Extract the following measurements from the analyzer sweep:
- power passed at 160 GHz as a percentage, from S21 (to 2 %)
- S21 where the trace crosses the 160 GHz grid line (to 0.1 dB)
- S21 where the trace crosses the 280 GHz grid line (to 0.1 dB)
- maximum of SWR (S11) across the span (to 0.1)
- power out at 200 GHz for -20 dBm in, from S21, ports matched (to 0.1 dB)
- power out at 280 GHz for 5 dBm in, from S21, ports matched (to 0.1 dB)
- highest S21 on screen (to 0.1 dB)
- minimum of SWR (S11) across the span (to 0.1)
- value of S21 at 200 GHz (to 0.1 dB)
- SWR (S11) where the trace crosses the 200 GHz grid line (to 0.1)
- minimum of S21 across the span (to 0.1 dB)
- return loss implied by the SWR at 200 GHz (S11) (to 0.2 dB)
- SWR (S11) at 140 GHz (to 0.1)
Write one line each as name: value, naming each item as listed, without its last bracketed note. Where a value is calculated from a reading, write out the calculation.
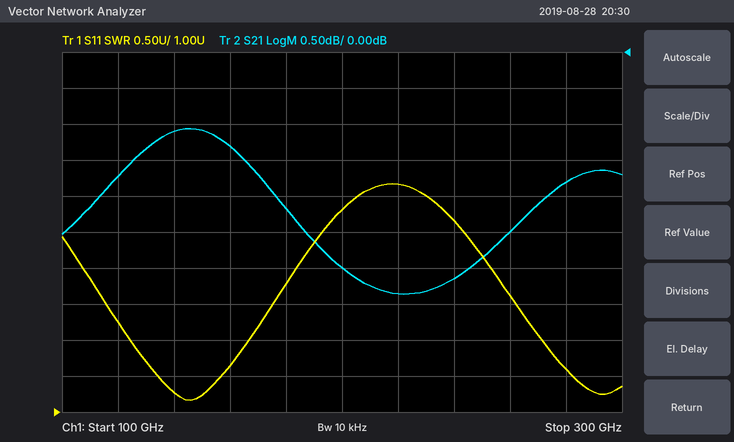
power passed at 160 GHz as a percentage, from S21: 10^(-1.3/10) ≈ 74 %
S21 where the trace crosses the 160 GHz grid line: -1.3 dB
S21 where the trace crosses the 280 GHz grid line: -1.8 dB
maximum of SWR (S11) across the span: 4.2
power out at 200 GHz for -20 dBm in, from S21, ports matched: -20 dBm + (-3.0 dB) = -23.0 dBm
power out at 280 GHz for 5 dBm in, from S21, ports matched: 5 dBm + (-1.8 dB) = 3.2 dBm
highest S21 on screen: -1.1 dB
minimum of SWR (S11) across the span: 1.2
value of S21 at 200 GHz: -3.0 dB
SWR (S11) where the trace crosses the 200 GHz grid line: 3.8
minimum of S21 across the span: -3.4 dB
return loss implied by the SWR at 200 GHz (S11): −20 log10((3.8 − 1)/(3.8 + 1)) ≈ 4.68 dB, so 4.6 dB to the nearest 0.2 dB
SWR (S11) at 140 GHz: 1.3
